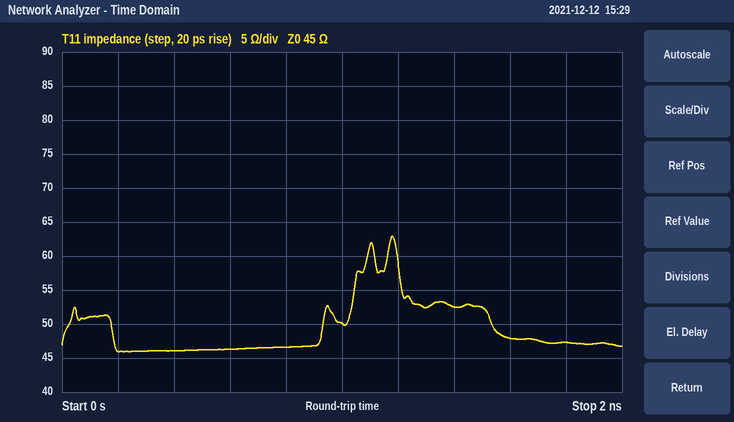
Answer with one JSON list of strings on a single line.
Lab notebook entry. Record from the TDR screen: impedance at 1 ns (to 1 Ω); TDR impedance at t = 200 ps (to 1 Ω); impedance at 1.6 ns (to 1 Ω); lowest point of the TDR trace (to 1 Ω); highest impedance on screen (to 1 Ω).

["50 Ω", "46 Ω", "48 Ω", "46 Ω", "63 Ω"]
